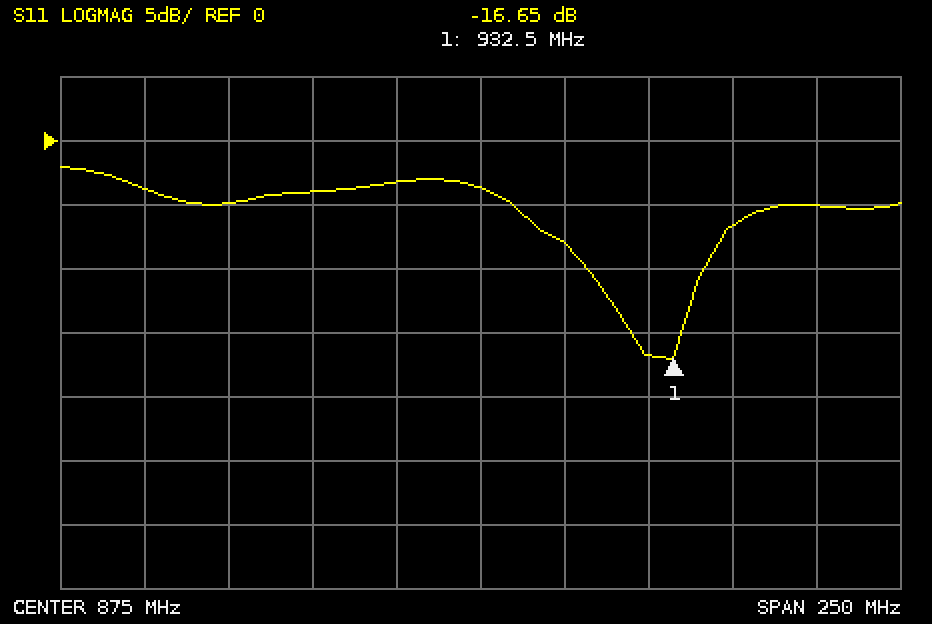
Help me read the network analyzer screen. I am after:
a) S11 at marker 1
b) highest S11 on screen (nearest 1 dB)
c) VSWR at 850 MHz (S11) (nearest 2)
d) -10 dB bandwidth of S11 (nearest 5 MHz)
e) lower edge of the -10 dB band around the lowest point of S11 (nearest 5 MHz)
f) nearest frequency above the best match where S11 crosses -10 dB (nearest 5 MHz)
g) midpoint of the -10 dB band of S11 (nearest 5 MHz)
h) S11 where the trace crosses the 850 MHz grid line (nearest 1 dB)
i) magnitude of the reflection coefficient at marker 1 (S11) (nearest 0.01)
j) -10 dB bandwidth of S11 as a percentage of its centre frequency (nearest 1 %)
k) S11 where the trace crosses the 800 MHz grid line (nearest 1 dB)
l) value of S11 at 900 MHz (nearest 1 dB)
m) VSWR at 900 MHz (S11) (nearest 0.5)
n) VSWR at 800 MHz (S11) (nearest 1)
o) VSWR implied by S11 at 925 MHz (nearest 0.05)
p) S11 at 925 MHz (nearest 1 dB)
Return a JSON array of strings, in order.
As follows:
["-16.65 dB", "-2 dB", "6", "35 MHz", "905 MHz", "940 MHz", "925 MHz", "-3 dB", "0.15", "4 %", "-5 dB", "-8 dB", "2.5", "4", "1.35", "-17 dB"]
